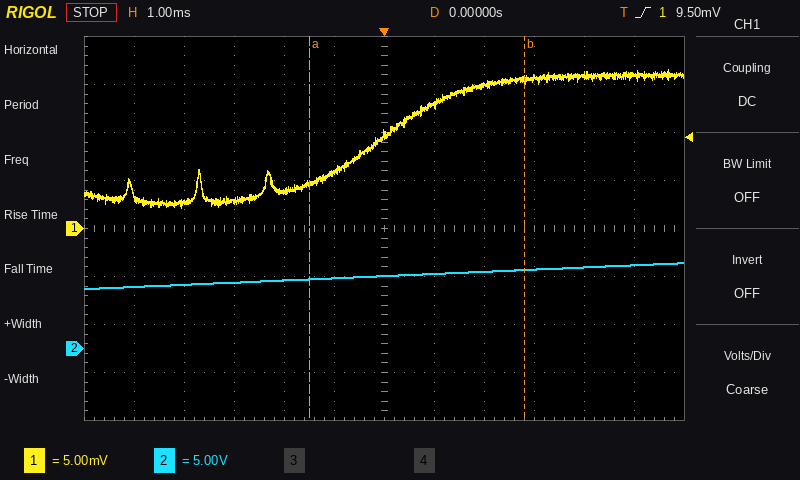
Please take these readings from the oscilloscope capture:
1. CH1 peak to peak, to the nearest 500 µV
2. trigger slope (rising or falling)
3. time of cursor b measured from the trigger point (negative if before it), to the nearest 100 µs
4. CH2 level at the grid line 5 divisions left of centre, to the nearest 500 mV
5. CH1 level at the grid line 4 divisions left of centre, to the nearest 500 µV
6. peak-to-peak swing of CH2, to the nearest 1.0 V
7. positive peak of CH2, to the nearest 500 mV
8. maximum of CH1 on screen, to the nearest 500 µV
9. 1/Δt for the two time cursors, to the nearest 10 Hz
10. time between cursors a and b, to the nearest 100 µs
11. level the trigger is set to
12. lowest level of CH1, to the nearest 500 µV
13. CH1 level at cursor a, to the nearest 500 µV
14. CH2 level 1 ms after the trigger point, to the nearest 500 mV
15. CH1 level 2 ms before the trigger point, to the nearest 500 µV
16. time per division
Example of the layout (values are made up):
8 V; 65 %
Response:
14.5 mV; rising; +2.8 ms; 6.5 V; 2.5 mV; 3.0 V; 9.0 V; 16.5 mV; 230 Hz; 4.3 ms; 9.50 mV; 2.0 mV; 4.5 mV; 8.0 V; 4.0 mV; 1 ms
